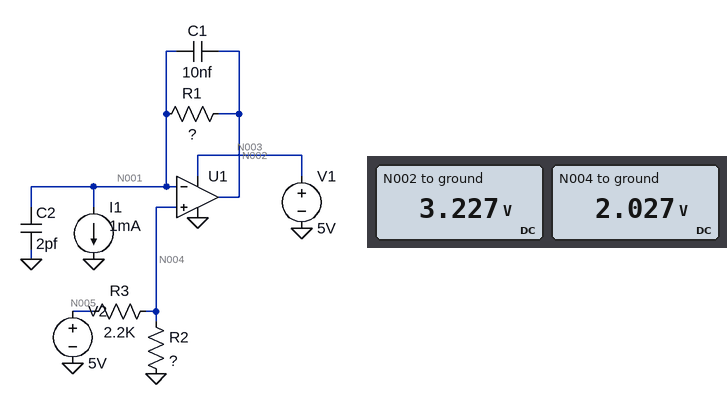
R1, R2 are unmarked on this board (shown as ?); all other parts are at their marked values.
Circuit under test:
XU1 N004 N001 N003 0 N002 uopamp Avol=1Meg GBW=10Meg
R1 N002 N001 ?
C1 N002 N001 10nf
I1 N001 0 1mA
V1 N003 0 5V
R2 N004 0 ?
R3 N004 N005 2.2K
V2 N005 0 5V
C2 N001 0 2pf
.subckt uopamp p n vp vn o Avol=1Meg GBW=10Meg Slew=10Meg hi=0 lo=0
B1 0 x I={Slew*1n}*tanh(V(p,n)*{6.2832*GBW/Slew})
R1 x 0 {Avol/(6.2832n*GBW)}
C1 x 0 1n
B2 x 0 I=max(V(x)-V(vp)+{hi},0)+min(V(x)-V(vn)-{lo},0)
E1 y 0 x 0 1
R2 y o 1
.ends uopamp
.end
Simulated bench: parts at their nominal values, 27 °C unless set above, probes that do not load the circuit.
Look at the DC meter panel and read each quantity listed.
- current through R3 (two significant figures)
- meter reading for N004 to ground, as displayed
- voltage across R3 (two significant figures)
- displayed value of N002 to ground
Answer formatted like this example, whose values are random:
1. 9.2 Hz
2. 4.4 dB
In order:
1. 1.4 mA
2. 2.027 V
3. 3.0 V
4. 3.227 V
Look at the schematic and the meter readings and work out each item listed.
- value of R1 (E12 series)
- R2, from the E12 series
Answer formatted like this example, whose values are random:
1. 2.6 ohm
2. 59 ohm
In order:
1. 1.2 kΩ
2. 1.5 kΩ
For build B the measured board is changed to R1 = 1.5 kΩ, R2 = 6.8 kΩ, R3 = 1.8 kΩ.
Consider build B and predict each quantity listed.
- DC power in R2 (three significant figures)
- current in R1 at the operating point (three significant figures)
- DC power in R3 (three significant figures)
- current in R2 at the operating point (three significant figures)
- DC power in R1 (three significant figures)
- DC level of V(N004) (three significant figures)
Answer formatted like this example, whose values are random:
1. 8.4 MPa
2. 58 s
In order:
1. 2.30 mW
2. 1.00 mA
3. 608 µW
4. 581 µA
5. 1.50 mW
6. 3.95 V
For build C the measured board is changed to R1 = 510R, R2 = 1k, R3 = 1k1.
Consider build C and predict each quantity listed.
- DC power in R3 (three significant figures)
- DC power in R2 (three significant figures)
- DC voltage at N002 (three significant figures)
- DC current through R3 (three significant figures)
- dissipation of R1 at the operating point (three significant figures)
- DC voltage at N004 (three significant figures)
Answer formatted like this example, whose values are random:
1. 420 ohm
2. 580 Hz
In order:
1. 6.24 mW
2. 5.67 mW
3. 2.89 V
4. 2.38 mA
5. 510 µW
6. 2.38 V
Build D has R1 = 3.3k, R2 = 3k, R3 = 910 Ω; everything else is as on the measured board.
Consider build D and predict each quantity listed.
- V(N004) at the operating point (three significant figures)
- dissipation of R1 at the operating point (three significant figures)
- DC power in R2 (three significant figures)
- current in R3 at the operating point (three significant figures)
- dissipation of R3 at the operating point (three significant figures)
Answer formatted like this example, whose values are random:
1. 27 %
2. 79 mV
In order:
1. 3.84 V
2. 3.30 mW
3. 4.91 mW
4. 1.28 mA
5. 1.49 mW
